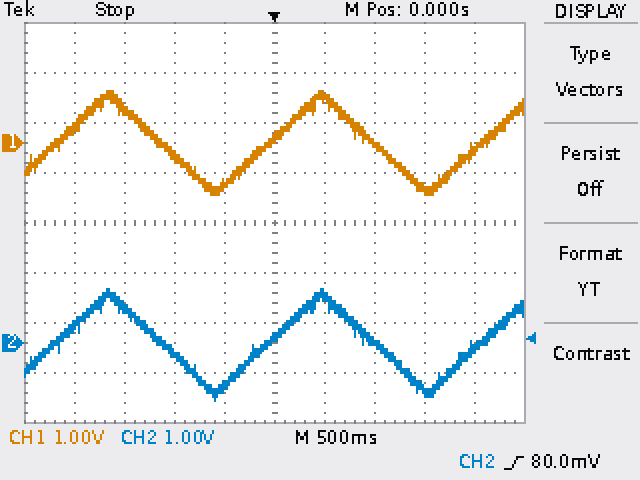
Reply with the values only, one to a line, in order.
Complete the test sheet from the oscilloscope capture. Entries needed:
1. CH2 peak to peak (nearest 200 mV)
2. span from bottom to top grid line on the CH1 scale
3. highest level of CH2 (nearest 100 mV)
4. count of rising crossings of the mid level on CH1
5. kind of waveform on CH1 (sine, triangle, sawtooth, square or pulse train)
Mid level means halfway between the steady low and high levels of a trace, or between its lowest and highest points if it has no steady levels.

2.2 V
8 V
1.1 V
3
triangle
